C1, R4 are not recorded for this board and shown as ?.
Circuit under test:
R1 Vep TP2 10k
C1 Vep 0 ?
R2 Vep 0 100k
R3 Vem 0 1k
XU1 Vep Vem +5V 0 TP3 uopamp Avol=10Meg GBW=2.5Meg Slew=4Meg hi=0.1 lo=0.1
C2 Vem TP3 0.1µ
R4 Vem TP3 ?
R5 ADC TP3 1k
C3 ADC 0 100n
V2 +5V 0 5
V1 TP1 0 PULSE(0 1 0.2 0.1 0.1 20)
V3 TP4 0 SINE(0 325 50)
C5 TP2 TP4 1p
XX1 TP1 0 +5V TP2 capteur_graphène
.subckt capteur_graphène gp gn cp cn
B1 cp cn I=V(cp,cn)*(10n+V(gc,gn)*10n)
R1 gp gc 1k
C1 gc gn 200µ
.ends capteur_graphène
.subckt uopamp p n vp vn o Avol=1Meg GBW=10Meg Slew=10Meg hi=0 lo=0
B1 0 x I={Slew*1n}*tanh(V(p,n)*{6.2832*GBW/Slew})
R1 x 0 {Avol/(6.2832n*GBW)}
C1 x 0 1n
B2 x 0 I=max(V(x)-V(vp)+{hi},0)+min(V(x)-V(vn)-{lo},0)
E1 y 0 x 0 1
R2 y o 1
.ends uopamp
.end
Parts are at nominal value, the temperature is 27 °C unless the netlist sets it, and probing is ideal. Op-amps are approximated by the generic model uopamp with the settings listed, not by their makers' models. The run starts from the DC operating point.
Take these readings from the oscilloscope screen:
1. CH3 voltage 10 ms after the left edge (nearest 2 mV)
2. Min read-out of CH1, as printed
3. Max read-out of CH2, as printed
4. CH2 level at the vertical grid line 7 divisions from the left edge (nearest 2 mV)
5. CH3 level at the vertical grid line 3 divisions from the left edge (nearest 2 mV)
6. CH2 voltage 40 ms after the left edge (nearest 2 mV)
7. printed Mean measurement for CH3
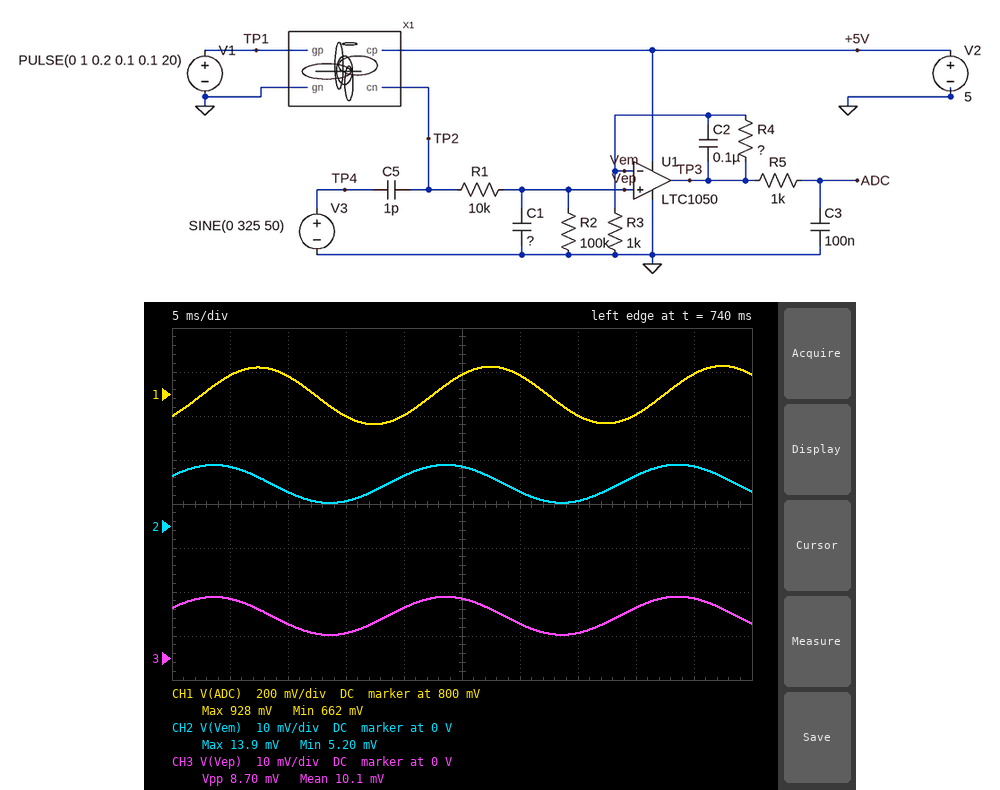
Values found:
8 mV
662 mV
13.9 mV
6 mV
6 mV
12 mV
10.1 mV
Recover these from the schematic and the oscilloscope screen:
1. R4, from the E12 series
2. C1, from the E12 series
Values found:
82 kΩ
68 nF
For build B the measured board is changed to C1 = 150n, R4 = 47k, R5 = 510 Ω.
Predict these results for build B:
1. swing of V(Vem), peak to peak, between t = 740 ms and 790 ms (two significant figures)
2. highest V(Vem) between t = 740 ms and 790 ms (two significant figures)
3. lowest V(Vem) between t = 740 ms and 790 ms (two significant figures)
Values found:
4.3 mV
12 mV
7.4 mV
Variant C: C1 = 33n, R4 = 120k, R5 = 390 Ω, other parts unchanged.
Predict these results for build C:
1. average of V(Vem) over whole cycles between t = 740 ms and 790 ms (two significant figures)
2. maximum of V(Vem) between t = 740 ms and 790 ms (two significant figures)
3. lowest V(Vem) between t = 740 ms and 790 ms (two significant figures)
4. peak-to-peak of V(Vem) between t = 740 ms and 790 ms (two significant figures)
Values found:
9.6 mV
17 mV
2.5 mV
14 mV
